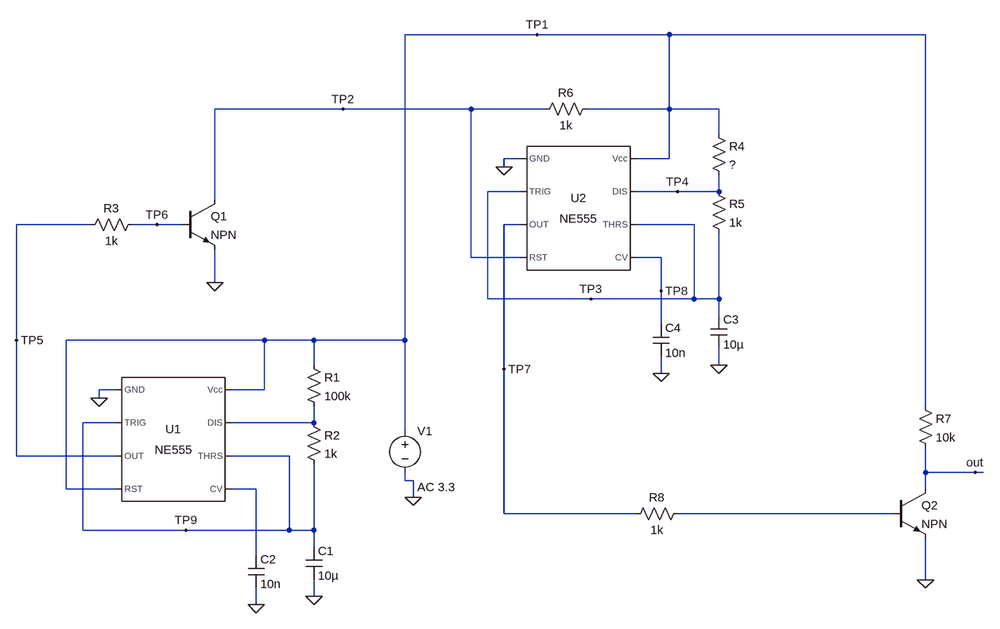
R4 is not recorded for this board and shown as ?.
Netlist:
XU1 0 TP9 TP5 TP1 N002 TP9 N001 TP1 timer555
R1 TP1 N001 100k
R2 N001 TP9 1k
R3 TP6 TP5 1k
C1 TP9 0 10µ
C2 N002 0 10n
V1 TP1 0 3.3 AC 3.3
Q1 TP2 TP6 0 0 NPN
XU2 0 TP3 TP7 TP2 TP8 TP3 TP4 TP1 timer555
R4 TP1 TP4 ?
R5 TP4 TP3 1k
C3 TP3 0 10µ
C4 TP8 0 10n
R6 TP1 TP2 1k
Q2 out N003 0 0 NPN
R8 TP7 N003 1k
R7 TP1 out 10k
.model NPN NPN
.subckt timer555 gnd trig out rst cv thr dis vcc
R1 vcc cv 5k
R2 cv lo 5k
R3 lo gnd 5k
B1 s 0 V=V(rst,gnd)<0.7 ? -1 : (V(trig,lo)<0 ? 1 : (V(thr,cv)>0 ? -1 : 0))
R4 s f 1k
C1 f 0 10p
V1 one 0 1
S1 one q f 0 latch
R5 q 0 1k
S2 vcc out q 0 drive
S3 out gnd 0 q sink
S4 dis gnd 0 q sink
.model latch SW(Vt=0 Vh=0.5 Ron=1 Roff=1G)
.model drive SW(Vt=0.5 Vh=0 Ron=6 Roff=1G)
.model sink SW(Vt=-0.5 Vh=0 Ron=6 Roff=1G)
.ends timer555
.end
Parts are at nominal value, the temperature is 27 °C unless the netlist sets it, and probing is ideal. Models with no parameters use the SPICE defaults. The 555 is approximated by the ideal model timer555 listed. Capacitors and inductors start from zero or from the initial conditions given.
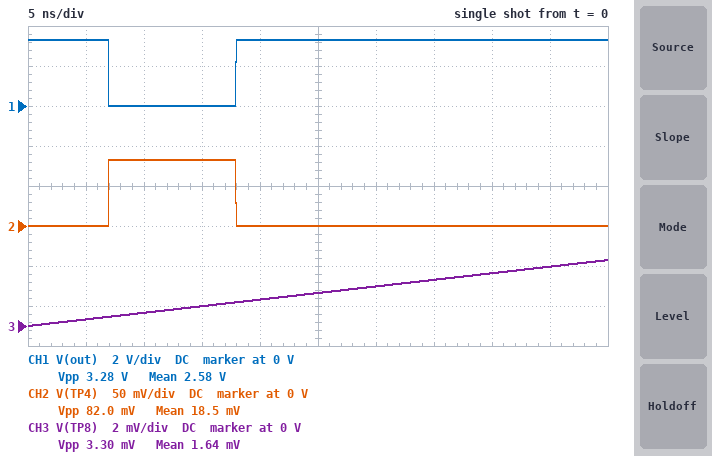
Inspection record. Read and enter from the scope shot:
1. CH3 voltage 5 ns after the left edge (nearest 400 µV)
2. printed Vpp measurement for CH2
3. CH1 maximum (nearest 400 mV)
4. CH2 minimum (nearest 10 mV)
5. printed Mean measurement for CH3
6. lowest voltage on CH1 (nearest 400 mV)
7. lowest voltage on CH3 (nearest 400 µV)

400 µV
82.0 mV
3.2 V
0 V
1.64 mV
0 V
0 V
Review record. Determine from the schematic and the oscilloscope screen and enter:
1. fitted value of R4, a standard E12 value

39 kΩ
